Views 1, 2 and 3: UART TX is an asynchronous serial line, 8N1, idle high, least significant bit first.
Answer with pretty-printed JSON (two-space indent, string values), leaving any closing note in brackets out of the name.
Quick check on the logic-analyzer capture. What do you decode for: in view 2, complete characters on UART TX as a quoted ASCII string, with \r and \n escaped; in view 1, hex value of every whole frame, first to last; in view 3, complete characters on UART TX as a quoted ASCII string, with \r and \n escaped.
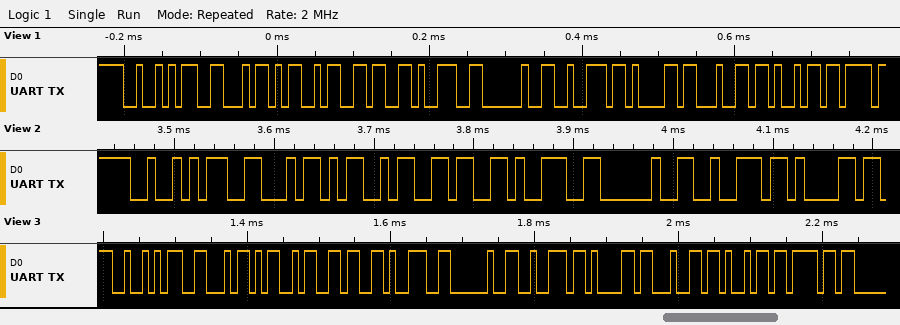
{
  "in view 2, complete characters on UART TX as a quoted ASCII string, with \\r and \\n escaped": "\"RFM69 ra\"",
  "in view 1, hex value of every whole frame, first to last": "52 46 4D 36 39 20 72 61 64 69",
  "in view 3, complete characters on UART TX as a quoted ASCII string, with \\r and \\n escaped": "\"RFM69 radio\""
}
